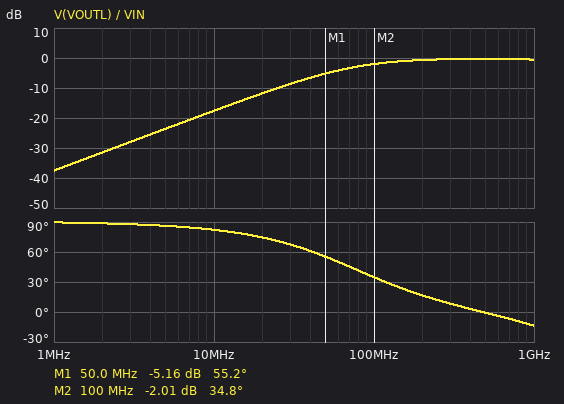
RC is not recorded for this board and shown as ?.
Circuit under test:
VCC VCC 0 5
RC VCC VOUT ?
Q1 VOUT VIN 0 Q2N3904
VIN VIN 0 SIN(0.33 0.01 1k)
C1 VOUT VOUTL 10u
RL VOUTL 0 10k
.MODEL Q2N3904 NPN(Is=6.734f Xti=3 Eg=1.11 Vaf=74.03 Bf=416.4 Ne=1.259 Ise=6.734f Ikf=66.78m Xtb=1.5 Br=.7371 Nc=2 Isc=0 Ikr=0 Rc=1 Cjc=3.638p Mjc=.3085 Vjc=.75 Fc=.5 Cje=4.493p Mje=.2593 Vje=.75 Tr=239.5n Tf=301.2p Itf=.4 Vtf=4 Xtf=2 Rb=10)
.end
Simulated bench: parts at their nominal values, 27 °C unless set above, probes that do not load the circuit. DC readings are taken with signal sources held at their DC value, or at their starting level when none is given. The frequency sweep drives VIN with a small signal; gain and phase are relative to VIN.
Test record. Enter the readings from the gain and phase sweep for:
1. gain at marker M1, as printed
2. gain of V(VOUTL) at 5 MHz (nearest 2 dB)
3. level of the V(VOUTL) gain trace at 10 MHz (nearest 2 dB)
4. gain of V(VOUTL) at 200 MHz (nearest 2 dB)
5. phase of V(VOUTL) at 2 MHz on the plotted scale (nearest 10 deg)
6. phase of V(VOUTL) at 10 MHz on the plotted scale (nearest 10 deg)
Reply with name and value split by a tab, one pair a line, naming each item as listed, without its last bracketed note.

gain at marker M1, as printed	-5.16 dB
gain of V(VOUTL) at 5 MHz	-24 dB
level of the V(VOUTL) gain trace at 10 MHz	-18 dB
gain of V(VOUTL) at 200 MHz	0 dB
phase of V(VOUTL) at 2 MHz on the plotted scale	90 deg
phase of V(VOUTL) at 10 MHz on the plotted scale	80 deg
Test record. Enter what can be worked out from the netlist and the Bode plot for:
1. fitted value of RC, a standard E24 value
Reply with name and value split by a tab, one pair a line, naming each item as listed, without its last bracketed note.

fitted value of RC, a standard E24 value	1.2 kΩ
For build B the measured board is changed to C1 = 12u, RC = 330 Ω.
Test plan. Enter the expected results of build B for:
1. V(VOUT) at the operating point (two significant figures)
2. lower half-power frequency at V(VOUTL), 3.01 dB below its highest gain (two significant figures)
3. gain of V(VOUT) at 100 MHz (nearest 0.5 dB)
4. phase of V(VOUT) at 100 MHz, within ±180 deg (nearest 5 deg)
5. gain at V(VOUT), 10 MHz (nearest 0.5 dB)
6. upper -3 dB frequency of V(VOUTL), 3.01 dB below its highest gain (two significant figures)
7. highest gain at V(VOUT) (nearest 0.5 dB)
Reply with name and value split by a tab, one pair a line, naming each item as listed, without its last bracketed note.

V(VOUT) at the operating point	5.0 V
lower half-power frequency at V(VOUTL), 3.01 dB below its highest gain	210 MHz
gain of V(VOUT) at 100 MHz	-8.5 dB
phase of V(VOUT) at 100 MHz, within ±180 deg	65 deg
gain at V(VOUT), 10 MHz	-28.0 dB
upper -3 dB frequency of V(VOUTL), 3.01 dB below its highest gain	3.6 GHz
highest gain at V(VOUT)	-1.0 dB
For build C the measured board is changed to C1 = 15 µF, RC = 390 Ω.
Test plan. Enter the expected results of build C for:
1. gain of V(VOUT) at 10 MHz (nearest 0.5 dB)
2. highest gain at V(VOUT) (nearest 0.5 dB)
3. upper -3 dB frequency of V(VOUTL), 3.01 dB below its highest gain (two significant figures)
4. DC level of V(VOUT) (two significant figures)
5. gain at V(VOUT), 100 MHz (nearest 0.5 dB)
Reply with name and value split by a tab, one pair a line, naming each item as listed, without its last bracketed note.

gain of V(VOUT) at 10 MHz	-26.5 dB
highest gain at V(VOUT)	-1.0 dB
upper -3 dB frequency of V(VOUTL), 3.01 dB below its highest gain	3.5 GHz
DC level of V(VOUT)	5.0 V
gain at V(VOUT), 100 MHz	-7.5 dB
